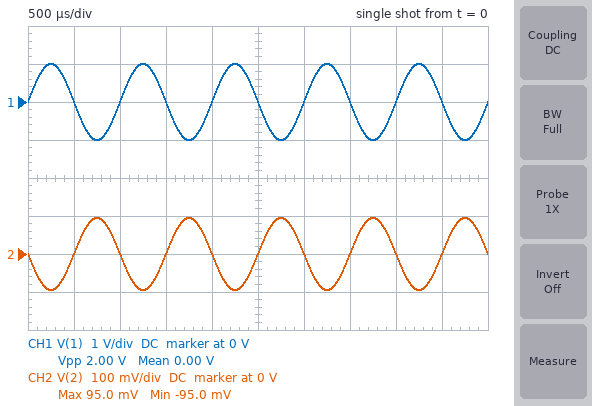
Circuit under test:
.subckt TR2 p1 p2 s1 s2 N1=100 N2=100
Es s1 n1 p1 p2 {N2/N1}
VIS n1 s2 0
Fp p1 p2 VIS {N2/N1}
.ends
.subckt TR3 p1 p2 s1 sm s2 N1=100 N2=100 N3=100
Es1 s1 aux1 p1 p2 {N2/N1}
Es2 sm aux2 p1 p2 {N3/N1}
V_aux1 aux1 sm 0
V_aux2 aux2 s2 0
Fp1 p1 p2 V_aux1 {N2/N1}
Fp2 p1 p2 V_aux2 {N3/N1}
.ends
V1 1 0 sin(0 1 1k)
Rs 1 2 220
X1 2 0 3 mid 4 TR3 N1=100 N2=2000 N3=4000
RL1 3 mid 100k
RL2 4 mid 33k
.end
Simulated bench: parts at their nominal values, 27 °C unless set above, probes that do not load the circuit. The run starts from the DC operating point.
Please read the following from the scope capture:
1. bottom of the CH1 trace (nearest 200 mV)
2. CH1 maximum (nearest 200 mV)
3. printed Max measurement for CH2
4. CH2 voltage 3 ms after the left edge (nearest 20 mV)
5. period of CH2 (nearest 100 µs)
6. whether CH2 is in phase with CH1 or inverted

-1.0 V
1.0 V
95.0 mV
0 V
1.0 ms
inverted
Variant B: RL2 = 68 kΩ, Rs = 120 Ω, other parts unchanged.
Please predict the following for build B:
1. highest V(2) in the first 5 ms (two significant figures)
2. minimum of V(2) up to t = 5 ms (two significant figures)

430 mV
-430 mV
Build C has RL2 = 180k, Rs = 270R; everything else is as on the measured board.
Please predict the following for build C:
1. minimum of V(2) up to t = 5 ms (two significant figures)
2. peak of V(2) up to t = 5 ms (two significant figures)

-400 mV
400 mV
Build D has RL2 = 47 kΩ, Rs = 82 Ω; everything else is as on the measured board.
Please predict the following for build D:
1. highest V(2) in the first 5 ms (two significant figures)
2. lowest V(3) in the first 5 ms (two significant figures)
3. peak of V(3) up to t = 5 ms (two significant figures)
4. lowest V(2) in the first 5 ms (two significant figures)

470 mV
-16 V
16 V
-470 mV
